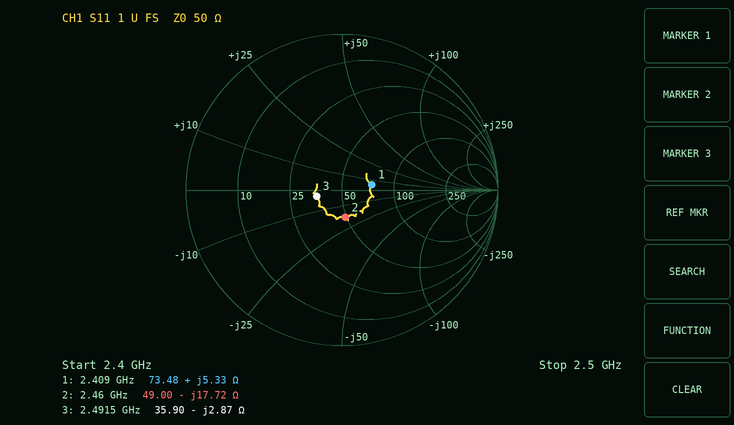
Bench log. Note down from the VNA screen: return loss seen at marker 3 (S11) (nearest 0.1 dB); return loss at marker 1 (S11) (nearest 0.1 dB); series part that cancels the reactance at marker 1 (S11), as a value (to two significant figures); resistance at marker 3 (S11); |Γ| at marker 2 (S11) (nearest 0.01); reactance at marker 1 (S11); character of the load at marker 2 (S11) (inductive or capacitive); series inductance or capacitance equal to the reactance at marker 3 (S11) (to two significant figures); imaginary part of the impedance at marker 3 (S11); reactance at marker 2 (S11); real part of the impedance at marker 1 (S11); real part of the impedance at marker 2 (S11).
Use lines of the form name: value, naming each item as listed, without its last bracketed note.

return loss seen at marker 3 (S11): 15.5 dB
return loss at marker 1 (S11): 14.2 dB
series part that cancels the reactance at marker 1 (S11), as a value: 12 pF
resistance at marker 3: 35.90 Ω
|Γ| at marker 2 (S11): 0.18
reactance at marker 1: +5.33 Ω
character of the load at marker 2 (S11): capacitive
series inductance or capacitance equal to the reactance at marker 3 (S11): 22 pF
imaginary part of the impedance at marker 3: -2.87 Ω
reactance at marker 2: -17.72 Ω
real part of the impedance at marker 1: 73.48 Ω
real part of the impedance at marker 2: 49.00 Ω
